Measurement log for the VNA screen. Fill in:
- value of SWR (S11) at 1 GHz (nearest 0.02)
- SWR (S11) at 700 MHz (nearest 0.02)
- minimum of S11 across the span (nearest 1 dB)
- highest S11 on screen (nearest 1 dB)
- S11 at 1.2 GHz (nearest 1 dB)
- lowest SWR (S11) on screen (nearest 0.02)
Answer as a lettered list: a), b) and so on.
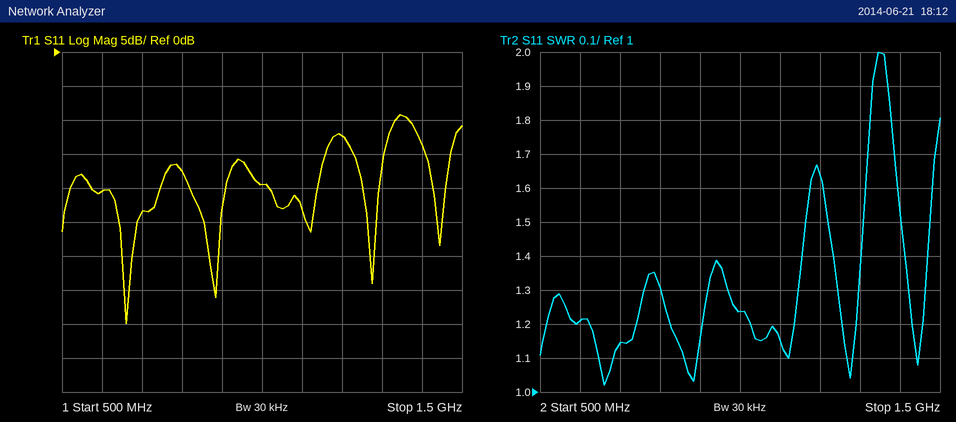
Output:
a) 1.24
b) 1.14
c) -40 dB
d) -9 dB
e) -12 dB
f) 1.02
